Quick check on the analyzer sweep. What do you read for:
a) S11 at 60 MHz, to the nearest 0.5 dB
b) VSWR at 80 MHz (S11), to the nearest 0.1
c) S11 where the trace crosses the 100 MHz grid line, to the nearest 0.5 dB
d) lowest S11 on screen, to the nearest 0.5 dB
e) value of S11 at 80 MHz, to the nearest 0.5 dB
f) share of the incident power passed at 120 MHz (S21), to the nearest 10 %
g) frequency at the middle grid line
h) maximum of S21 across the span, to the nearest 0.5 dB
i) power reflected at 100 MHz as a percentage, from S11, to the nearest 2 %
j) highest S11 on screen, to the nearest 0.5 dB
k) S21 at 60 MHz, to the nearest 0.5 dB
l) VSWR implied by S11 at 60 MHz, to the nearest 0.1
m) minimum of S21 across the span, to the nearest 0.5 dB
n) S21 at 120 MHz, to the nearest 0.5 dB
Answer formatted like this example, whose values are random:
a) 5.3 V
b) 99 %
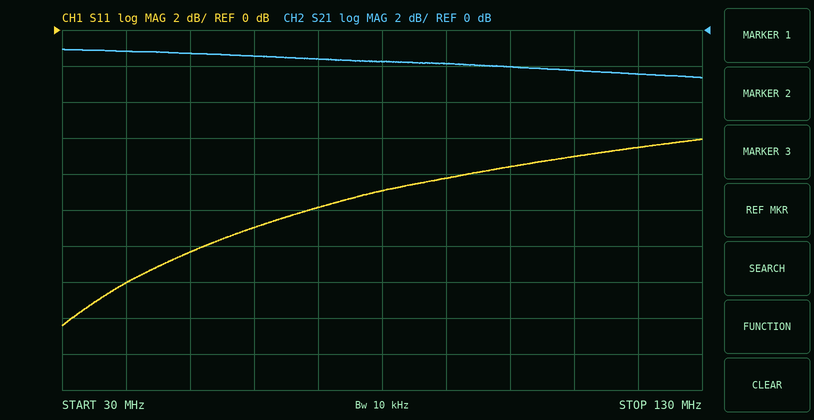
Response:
a) -11.0 dB
b) 2.1
c) -7.5 dB
d) -16.5 dB
e) -9.0 dB
f) 60 %
g) 80 MHz
h) -1.0 dB
i) 18 %
j) -6.0 dB
k) -1.5 dB
l) 1.8
m) -2.5 dB
n) -2.5 dB
